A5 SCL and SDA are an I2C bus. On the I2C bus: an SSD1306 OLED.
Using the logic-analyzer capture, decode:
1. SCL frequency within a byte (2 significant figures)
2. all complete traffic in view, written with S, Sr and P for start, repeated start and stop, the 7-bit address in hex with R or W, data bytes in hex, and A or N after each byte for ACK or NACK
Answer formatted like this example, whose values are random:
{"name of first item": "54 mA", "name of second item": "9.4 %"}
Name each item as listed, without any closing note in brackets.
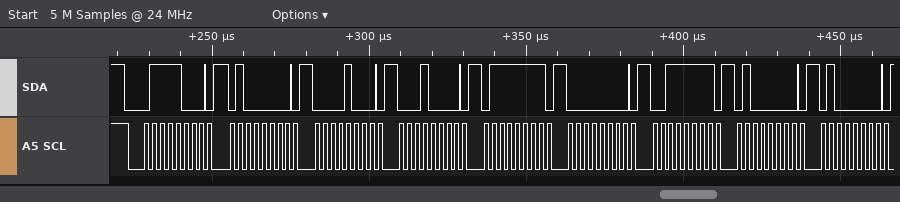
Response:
{"SCL frequency within a byte": "400 kHz", "all complete traffic in view, written with S, Sr and P for start, repeated start and stop, the 7-bit address in hex with R or W, data bytes in hex, and A or N after each byte for ACK or NACK": "S 3CW A 40 A 08 A 10 A 7F A 00 A 3F A 40 A 40 A"}
